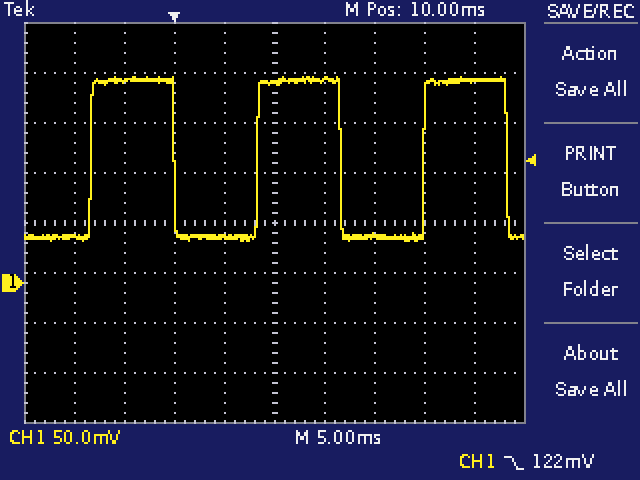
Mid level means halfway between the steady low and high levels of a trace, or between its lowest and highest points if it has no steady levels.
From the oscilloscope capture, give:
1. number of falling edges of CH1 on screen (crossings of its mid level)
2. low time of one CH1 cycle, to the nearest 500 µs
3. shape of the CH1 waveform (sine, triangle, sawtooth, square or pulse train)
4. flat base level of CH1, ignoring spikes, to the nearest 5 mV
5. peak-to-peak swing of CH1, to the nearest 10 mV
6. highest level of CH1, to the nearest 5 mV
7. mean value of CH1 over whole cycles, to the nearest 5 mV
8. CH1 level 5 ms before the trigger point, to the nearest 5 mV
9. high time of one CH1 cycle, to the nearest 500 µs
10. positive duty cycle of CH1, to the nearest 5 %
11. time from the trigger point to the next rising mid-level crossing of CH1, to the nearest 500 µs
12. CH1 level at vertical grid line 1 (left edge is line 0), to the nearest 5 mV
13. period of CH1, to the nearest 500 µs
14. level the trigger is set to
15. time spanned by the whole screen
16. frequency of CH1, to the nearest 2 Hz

3
8.5 ms
square
45 mV
160 mV
205 mV
125 mV
200 mV
8.5 ms
50 %
8.5 ms
45 mV
16.5 ms
122 mV
50 ms
60 Hz
